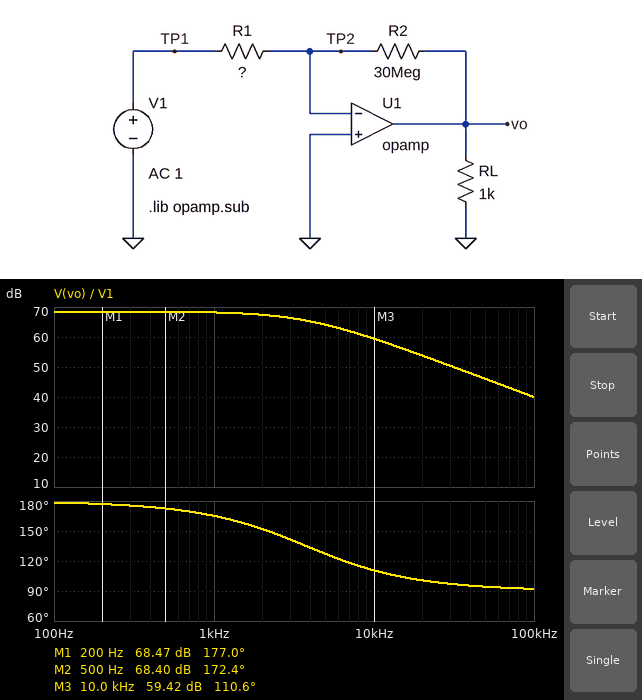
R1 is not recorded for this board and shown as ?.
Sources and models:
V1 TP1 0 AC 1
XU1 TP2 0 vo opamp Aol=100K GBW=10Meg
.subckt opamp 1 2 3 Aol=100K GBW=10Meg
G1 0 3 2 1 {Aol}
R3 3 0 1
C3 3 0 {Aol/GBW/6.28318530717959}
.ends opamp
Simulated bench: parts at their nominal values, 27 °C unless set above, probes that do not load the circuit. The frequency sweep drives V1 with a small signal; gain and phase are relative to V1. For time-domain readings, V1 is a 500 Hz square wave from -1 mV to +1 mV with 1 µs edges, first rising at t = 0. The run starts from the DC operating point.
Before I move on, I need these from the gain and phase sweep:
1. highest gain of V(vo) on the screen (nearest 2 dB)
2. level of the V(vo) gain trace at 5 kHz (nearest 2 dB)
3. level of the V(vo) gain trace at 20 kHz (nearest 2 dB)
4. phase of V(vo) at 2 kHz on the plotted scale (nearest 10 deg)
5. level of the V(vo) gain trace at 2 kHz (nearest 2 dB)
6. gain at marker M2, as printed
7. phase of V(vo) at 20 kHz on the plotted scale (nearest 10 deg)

68 dB
64 dB
54 dB
150 deg
68 dB
68.40 dB
100 deg
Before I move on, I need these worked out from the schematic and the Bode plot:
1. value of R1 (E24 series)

11 kΩ
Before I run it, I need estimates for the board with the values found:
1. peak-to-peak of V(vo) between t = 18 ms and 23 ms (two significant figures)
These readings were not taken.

5.3 V
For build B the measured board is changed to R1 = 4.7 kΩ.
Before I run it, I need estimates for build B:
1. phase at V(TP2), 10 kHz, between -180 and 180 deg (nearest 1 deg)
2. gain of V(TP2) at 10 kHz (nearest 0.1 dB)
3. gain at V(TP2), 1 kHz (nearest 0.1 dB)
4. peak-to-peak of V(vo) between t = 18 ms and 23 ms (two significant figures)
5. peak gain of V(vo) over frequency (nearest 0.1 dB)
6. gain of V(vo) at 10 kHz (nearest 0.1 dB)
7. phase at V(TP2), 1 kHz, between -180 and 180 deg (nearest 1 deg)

9 deg
-0.1 dB
-5.7 dB
12 V
75.6 dB
59.9 dB
53 deg
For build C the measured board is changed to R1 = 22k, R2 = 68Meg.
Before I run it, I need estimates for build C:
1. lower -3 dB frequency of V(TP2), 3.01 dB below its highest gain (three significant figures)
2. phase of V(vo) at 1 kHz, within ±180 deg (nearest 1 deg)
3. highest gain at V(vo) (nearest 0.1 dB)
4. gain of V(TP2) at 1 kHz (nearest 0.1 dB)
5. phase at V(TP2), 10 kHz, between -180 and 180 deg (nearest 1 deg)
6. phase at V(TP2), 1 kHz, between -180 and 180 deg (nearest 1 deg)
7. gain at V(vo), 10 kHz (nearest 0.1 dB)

3.33 kHz
163 deg
69.5 dB
-10.8 dB
18 deg
68 deg
59.5 dB
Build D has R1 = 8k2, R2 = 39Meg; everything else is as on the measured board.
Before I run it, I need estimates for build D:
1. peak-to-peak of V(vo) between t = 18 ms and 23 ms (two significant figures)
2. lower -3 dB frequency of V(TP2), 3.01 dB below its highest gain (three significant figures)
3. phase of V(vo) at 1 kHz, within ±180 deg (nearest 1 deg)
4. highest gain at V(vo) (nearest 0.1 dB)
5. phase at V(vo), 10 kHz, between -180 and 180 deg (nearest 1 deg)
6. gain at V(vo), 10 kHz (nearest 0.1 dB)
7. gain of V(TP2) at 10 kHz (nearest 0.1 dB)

9.1 V
2.20 kHz
156 deg
73.1 dB
102 deg
59.8 dB
-0.2 dB
